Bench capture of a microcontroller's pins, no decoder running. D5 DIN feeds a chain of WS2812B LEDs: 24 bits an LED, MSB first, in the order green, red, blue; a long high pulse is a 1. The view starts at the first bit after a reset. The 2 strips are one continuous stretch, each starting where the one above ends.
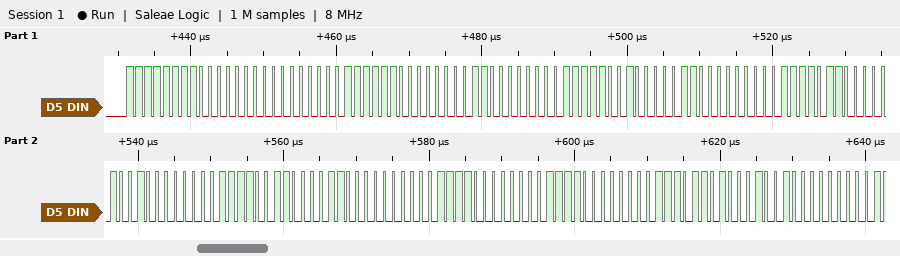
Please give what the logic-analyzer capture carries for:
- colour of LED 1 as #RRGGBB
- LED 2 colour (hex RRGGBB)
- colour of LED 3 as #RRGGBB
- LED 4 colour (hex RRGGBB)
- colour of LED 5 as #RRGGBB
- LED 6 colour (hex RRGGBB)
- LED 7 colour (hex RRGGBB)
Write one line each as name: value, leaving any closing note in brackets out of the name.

colour of LED 1 as #RRGGBB: #00FF00
LED 2 colour: #03FC00
colour of LED 3 as #RRGGBB: #06F900
LED 4 colour: #09F600
colour of LED 5 as #RRGGBB: #0CF300
LED 6 colour: #0FF000
LED 7 colour: #12ED00
